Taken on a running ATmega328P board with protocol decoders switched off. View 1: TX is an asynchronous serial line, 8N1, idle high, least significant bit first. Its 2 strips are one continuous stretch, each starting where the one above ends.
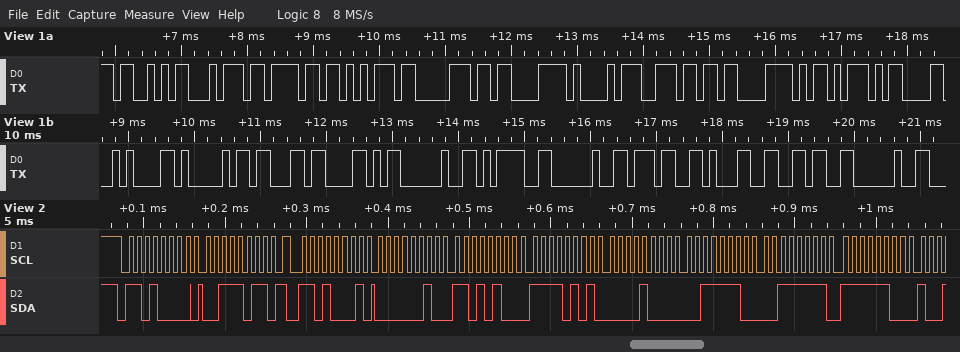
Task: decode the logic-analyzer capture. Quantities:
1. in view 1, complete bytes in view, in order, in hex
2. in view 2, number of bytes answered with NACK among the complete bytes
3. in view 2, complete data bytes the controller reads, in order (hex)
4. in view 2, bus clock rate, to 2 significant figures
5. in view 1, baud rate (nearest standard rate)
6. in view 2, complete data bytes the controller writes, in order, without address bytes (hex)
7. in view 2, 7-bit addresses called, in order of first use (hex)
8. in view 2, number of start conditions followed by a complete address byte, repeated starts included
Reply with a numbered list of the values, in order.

1. 53 74 6F 75 70 C3 A1 6E C3 AD 0D 0A 41 63 58 20 3D 20 37 31 36 20
2. 0
3. 02 D4 F5 08 3E 3F FC
4. 100 kHz
5. 9600 baud
6. 3B
7. 0x68
8. 2
